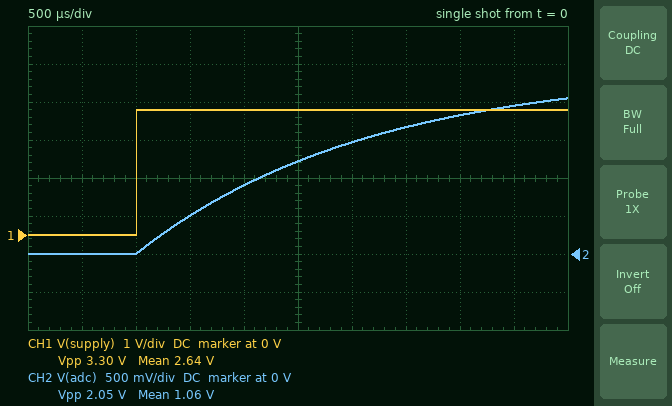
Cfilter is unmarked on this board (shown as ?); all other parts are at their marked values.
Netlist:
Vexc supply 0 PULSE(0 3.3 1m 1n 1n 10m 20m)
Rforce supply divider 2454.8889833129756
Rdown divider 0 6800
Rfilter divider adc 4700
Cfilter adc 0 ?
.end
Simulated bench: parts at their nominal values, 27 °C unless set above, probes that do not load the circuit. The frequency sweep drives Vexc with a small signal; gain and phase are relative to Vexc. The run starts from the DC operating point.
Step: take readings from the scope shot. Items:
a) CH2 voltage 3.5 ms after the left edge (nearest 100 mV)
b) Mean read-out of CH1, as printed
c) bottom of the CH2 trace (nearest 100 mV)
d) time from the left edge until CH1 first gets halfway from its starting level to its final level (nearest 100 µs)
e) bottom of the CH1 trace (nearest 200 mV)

1.7 V
2.64 V
0 V
1.0 ms
0 V
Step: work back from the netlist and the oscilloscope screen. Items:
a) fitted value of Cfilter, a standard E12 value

330 nF
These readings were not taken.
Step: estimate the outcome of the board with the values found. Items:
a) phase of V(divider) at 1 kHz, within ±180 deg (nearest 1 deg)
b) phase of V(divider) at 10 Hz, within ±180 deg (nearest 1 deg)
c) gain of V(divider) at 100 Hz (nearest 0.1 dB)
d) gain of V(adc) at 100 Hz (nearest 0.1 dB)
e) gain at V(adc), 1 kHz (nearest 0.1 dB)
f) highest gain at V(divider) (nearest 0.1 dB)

-2 deg
-2 deg
-4.3 dB
-7.2 dB
-25.3 dB
-2.7 dB
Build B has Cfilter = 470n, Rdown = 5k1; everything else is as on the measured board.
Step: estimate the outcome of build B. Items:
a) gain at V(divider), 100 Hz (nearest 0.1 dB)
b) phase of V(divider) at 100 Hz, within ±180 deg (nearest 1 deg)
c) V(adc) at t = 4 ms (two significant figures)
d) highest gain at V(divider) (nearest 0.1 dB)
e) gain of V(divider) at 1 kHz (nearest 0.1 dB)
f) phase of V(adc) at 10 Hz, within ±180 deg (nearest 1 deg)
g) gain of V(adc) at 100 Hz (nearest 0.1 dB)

-5.3 dB
-8 deg
1.4 V
-3.4 dB
-6.0 dB
-11 deg
-10.0 dB
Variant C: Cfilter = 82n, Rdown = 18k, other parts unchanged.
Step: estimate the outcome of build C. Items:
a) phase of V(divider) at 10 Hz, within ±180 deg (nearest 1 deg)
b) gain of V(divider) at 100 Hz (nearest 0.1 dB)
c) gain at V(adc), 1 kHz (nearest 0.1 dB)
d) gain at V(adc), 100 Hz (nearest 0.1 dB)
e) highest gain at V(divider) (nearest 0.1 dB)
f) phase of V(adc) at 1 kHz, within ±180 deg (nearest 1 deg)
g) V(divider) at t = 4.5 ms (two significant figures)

-1 deg
-1.4 dB
-12.4 dB
-1.6 dB
-1.1 dB
-74 deg
2.9 V
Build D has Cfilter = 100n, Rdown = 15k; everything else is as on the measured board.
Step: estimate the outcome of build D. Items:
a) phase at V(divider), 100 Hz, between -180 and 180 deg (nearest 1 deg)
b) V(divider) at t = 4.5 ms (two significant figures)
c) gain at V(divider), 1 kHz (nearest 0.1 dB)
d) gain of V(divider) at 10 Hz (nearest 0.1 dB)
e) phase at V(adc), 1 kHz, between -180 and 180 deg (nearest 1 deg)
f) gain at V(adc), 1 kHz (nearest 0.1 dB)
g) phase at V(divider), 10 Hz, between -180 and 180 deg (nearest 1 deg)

-7 deg
2.8 V
-4.3 dB
-1.3 dB
-77 deg
-14.2 dB
-1 deg
